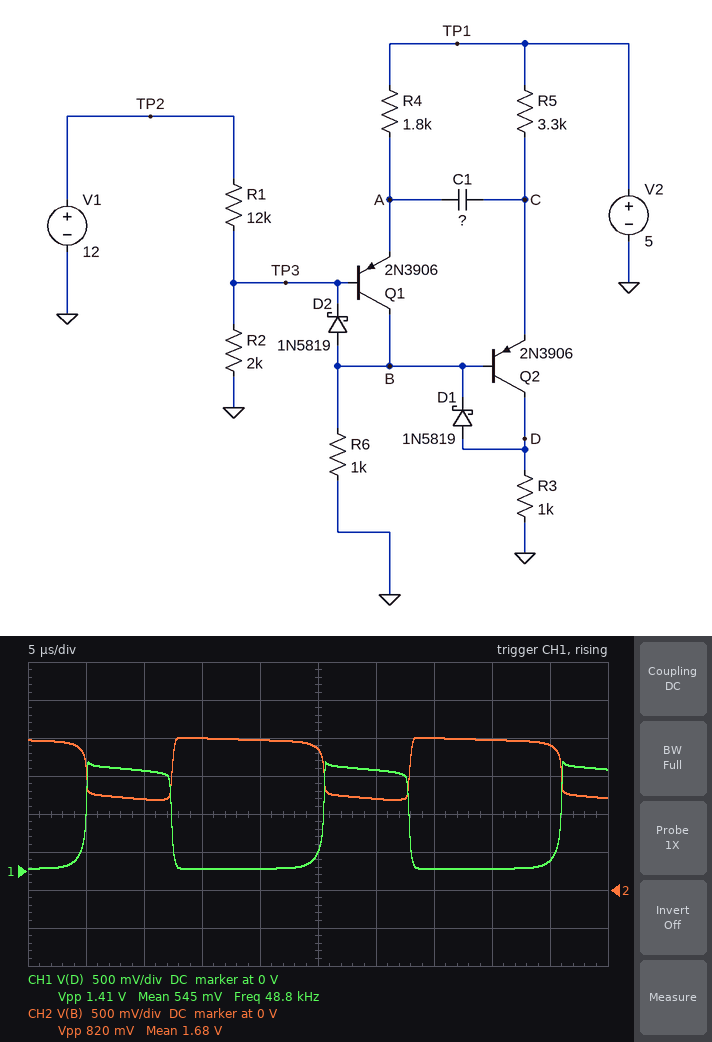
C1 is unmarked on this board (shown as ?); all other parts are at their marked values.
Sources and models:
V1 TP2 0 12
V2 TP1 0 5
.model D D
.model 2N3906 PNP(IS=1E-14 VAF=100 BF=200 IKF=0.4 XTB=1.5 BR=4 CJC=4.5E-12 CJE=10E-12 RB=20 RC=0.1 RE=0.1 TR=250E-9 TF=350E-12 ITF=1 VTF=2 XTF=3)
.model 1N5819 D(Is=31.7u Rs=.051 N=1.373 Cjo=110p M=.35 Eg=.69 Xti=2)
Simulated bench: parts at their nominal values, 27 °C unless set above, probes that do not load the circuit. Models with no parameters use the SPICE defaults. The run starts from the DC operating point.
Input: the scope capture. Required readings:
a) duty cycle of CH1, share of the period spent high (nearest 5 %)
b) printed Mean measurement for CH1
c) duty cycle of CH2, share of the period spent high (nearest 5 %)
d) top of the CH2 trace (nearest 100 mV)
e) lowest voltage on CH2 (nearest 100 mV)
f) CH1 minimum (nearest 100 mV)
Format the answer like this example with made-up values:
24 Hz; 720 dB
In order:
35 %; 545 mV; 65 %; 2.0 V; 1.2 V; 0 V
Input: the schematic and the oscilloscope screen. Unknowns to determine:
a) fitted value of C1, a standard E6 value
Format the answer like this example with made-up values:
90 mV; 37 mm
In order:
22 nF
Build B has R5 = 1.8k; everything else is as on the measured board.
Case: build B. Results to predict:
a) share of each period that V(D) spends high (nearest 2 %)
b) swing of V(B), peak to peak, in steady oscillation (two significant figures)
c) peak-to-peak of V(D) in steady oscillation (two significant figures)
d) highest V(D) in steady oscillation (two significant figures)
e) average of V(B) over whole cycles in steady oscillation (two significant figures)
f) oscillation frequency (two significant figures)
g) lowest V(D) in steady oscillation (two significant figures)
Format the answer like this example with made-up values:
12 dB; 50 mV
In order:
56 %; 720 mV; 1.6 V; 1.7 V; 1.8 V; 120 kHz; 33 mV
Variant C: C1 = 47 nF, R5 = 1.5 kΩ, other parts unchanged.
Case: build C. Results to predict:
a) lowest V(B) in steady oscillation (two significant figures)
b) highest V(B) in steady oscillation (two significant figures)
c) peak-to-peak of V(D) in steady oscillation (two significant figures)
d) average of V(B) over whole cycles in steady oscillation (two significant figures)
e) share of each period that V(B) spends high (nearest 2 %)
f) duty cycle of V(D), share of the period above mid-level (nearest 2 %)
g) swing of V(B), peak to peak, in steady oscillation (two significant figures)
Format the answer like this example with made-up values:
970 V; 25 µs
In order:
1.6 V; 2.3 V; 1.7 V; 1.8 V; 34 %; 66 %; 670 mV
